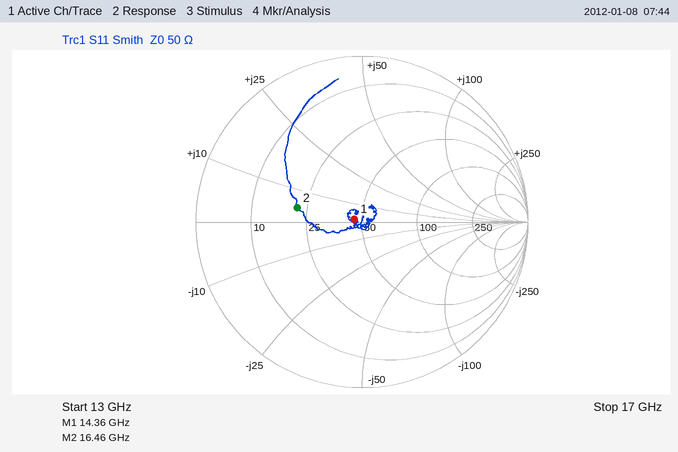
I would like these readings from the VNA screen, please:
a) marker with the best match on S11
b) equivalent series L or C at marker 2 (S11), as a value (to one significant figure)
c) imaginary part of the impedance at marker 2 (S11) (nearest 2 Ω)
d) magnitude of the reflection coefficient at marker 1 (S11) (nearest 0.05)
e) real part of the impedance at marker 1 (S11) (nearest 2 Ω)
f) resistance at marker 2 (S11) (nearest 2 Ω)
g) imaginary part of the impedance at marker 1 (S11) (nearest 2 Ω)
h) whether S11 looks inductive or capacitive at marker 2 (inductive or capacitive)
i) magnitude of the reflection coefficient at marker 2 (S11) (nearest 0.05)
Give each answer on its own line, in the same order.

marker 1
40 pH
+4 Ω
0.05
46 Ω
22 Ω
+2 Ω
inductive
0.40
